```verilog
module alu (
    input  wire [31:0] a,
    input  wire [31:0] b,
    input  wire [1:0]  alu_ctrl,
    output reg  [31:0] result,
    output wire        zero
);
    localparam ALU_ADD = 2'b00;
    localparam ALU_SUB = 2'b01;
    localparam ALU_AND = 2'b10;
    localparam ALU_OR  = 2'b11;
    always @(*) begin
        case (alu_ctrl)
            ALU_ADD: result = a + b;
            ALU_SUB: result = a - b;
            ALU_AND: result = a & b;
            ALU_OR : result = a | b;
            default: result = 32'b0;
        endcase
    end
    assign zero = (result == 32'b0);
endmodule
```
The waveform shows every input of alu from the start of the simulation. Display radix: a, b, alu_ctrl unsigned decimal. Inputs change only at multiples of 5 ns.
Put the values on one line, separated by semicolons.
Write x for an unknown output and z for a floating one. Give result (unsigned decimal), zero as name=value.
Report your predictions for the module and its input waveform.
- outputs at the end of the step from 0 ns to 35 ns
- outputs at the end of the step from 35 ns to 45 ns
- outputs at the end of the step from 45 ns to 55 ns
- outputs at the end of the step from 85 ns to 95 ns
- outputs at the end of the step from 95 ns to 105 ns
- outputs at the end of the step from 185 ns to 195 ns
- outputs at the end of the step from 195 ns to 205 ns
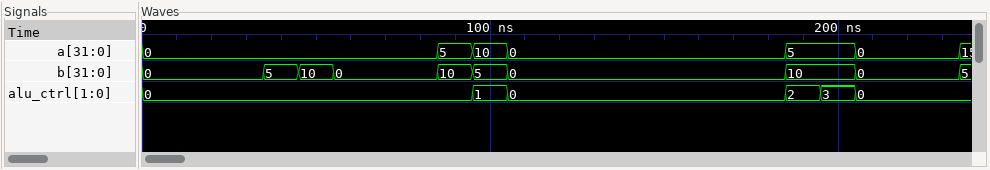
result=0, zero=1; result=5, zero=0; result=10, zero=0; result=15, zero=0; result=5, zero=0; result=0, zero=1; result=15, zero=0
